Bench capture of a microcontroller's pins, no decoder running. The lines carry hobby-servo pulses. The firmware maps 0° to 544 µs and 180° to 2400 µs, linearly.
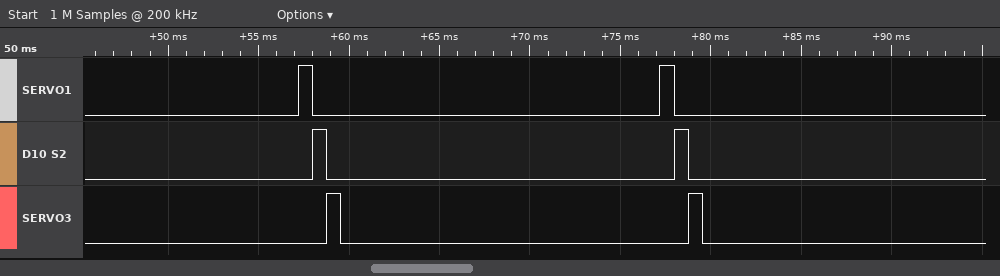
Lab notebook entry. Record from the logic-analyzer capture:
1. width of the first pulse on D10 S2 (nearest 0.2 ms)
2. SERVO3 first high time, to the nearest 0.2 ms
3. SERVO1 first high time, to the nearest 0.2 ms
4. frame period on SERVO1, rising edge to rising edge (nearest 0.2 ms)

0.8 ms
0.8 ms
0.8 ms
20.0 ms
